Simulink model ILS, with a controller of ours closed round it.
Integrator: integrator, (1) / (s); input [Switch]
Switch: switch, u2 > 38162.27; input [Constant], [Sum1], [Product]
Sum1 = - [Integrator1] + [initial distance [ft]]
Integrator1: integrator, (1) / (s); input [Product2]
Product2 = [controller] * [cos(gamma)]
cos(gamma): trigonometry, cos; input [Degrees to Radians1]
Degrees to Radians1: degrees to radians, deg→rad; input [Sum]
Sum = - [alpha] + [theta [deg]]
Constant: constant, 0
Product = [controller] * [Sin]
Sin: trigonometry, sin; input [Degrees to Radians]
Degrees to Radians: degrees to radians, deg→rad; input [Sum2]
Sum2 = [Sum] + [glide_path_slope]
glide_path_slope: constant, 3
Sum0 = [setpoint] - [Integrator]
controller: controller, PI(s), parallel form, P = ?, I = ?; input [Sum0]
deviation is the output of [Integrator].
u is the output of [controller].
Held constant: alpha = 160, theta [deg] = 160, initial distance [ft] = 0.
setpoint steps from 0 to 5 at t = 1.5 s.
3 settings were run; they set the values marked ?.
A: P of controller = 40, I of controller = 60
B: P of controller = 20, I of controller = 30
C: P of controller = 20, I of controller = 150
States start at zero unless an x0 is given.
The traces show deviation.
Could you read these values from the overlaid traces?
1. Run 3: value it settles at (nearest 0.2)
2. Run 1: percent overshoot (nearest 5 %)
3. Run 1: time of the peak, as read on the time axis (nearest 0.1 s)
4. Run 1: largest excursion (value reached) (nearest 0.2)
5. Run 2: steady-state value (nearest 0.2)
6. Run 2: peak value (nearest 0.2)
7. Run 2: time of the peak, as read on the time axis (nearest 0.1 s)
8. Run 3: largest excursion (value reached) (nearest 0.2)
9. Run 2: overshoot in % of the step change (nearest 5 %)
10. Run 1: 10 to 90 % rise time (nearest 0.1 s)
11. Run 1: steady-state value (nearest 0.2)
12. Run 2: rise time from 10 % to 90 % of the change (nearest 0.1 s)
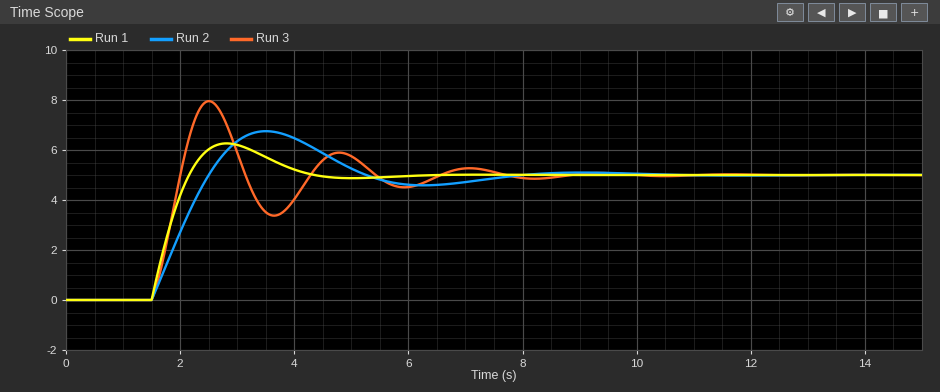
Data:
5.0
25 %
2.8 s
6.2
5.0
6.8
3.5 s
8.0
35 %
0.5 s
5.0
0.8 s
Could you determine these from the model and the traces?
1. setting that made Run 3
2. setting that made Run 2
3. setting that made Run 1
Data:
C
B
A
